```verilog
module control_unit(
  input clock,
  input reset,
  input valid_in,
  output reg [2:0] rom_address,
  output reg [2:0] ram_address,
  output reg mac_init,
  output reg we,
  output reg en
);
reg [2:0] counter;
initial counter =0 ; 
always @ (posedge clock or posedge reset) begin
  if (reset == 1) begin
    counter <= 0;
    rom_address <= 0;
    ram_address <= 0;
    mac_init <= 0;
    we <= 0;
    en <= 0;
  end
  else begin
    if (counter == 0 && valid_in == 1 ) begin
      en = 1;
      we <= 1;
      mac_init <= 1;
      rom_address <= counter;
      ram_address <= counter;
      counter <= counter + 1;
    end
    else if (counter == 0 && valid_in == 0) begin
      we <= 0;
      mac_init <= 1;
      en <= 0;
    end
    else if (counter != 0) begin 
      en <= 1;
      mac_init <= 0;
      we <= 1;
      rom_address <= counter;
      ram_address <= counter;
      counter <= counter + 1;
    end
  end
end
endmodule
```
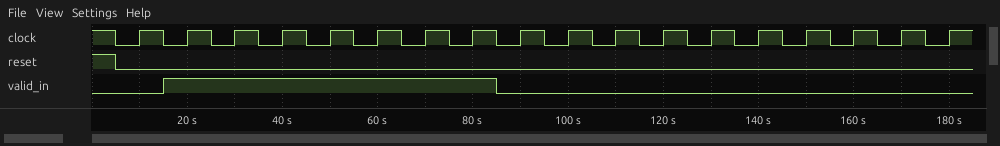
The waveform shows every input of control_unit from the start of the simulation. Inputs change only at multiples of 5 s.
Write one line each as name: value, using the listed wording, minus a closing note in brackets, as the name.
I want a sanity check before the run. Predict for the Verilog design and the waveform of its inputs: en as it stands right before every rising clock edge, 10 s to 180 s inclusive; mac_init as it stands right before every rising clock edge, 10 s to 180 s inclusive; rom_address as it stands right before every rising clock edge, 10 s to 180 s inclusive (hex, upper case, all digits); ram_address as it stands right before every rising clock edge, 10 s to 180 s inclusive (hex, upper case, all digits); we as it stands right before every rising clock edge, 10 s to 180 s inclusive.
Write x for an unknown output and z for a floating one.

en as it stands right before every rising clock edge, 10 s to 180 s inclusive: 0 0 1 1 1 1 1 1 1 1 0 0 0 0 0 0 0 0
mac_init as it stands right before every rising clock edge, 10 s to 180 s inclusive: 0 1 1 0 0 0 0 0 0 0 1 1 1 1 1 1 1 1
rom_address as it stands right before every rising clock edge, 10 s to 180 s inclusive: 0, 0, 0, 1, 2, 3, 4, 5, 6, 7, 7, 7, 7, 7, 7, 7, 7, 7
ram_address as it stands right before every rising clock edge, 10 s to 180 s inclusive: 0, 0, 0, 1, 2, 3, 4, 5, 6, 7, 7, 7, 7, 7, 7, 7, 7, 7
we as it stands right before every rising clock edge, 10 s to 180 s inclusive: 0 0 1 1 1 1 1 1 1 1 0 0 0 0 0 0 0 0
